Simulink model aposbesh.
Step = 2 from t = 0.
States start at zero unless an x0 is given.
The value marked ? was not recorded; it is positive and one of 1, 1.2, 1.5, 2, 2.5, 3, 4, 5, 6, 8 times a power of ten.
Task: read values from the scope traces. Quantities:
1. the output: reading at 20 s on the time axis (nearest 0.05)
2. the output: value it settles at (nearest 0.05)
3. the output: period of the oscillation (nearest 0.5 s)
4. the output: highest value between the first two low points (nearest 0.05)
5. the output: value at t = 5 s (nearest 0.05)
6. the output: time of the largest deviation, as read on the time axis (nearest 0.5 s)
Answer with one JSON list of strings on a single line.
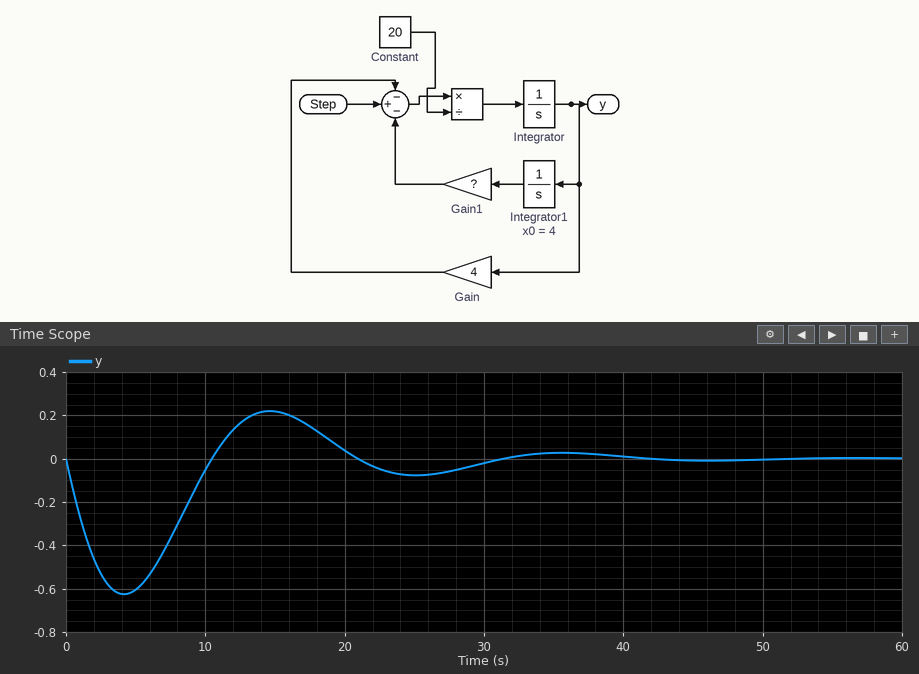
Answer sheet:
["0.05", "0.00", "21.0 s", "0.20", "-0.60", "4.0 s"]
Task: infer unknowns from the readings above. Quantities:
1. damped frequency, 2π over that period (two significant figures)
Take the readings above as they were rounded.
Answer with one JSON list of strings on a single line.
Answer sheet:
["0.30 rad/s"]
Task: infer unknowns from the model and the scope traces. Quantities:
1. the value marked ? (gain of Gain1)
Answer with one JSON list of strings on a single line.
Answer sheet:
["2"]
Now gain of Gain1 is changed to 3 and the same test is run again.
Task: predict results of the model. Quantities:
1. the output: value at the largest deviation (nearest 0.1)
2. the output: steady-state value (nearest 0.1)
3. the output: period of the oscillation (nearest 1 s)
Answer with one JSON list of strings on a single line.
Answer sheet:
["-0.9", "0.0", "17 s"]
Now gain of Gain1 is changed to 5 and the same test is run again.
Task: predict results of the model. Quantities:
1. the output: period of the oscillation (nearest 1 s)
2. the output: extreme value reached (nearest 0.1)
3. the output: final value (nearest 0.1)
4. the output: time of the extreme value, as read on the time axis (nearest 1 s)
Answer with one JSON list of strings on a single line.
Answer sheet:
["13 s", "-1.4", "0.0", "3 s"]
